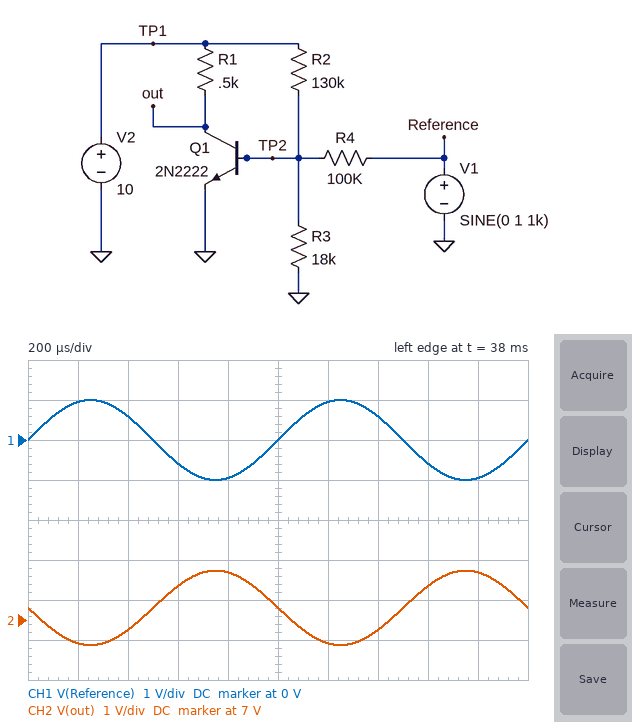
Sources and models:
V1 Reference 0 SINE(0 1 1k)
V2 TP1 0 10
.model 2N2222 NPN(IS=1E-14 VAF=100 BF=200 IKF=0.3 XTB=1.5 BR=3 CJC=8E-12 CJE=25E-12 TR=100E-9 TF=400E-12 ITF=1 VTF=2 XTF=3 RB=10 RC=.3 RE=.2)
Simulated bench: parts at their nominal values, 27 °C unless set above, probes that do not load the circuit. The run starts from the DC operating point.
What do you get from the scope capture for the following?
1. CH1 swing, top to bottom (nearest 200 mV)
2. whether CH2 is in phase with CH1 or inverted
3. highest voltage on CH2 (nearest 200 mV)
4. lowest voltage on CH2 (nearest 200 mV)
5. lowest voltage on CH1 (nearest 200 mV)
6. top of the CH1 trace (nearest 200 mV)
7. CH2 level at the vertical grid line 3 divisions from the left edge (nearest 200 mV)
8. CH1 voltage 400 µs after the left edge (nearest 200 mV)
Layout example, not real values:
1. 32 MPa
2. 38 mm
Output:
1. 2.0 V
2. inverted
3. 8.2 V
4. 6.4 V
5. -1.0 V
6. 1.0 V
7. 7.8 V
8. 600 mV
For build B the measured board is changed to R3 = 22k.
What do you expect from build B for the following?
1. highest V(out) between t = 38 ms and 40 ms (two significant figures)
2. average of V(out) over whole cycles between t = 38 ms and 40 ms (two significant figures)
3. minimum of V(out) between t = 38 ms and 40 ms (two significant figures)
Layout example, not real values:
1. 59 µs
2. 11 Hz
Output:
1. 7.6 V
2. 6.6 V
3. 5.7 V
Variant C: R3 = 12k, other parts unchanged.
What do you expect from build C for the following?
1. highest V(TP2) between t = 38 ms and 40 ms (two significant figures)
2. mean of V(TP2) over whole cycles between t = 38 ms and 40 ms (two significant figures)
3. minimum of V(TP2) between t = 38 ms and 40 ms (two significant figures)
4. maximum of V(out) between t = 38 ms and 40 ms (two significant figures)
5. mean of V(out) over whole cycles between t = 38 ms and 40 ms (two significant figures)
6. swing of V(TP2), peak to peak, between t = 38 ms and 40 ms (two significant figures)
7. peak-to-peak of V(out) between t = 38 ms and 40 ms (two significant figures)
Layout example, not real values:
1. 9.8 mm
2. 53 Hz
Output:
1. 690 mV
2. 670 mV
3. 640 mV
4. 9.7 V
5. 9.0 V
6. 51 mV
7. 1.6 V
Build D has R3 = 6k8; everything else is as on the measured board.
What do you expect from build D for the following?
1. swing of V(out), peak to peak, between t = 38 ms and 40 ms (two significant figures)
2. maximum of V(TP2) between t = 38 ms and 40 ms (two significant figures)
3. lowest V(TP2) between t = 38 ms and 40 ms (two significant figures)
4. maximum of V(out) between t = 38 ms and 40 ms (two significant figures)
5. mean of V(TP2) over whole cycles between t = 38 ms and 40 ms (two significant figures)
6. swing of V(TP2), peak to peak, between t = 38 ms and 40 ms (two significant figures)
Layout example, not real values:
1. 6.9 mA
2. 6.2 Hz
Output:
1. 3.9 mV
2. 530 mV
3. 410 mV
4. 10 V
5. 470 mV
6. 120 mV
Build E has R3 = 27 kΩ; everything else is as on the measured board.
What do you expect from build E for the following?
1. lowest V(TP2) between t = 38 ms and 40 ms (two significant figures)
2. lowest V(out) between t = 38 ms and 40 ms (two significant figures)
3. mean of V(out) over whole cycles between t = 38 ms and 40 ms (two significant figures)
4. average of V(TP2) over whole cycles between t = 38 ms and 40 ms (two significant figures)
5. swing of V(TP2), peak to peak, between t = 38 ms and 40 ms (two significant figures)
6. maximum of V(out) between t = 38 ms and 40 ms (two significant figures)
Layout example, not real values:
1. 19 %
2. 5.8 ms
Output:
1. 700 mV
2. 5.2 V
3. 6.1 V
4. 710 mV
5. 14 mV
6. 7.0 V
